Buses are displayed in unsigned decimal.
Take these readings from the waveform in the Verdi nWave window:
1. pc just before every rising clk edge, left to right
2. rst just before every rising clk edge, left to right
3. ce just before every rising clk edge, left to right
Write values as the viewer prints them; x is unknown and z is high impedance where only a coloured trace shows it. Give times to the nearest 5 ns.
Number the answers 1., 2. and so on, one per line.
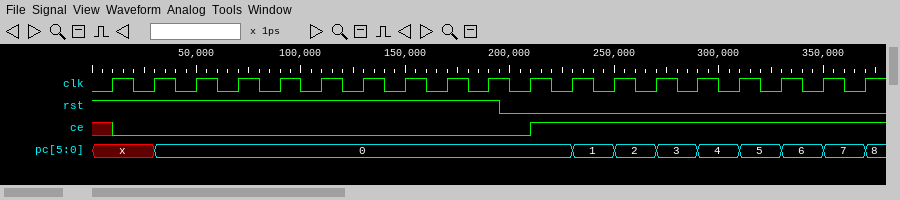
1. x, x, 0, 0, 0, 0, 0, 0, 0, 0, 0, 0, 1, 2, 3, 4, 5, 6, 7
2. 1 1 1 1 1 1 1 1 1 1 0 0 0 0 0 0 0 0 0
3. x 0 0 0 0 0 0 0 0 0 0 1 1 1 1 1 1 1 1
